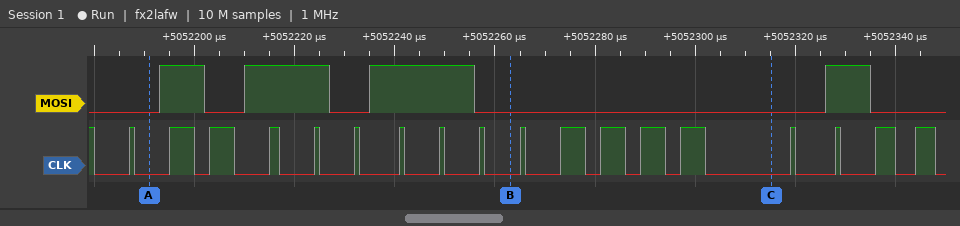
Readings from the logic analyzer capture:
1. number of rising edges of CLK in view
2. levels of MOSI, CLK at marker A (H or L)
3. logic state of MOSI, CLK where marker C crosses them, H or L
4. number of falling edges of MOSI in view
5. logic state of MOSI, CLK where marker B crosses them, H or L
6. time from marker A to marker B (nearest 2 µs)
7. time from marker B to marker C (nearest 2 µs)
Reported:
18
MOSI=L, CLK=L
MOSI=L, CLK=L
4
MOSI=L, CLK=L
72 µs
52 µs
